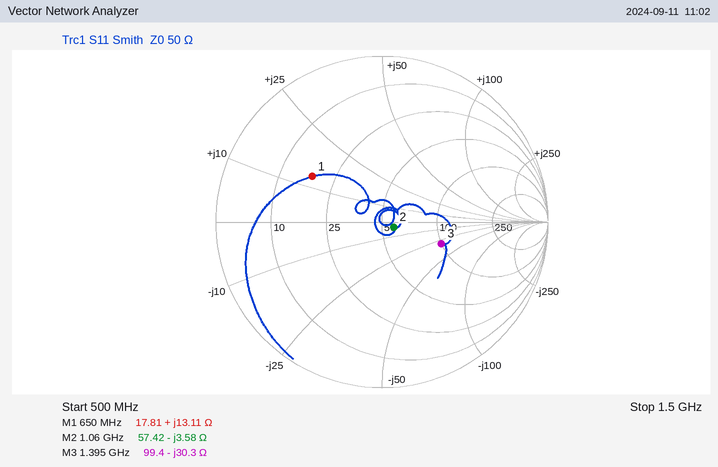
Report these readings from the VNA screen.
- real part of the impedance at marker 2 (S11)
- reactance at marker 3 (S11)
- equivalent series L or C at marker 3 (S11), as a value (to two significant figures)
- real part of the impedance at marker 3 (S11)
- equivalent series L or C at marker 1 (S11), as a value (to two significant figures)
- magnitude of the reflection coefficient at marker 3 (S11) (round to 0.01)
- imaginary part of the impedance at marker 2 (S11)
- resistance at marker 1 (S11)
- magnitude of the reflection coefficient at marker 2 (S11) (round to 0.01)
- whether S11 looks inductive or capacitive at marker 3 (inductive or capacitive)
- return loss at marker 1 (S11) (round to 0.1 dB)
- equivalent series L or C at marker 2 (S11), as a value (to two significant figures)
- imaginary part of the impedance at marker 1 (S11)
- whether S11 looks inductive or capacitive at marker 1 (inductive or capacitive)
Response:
57.42 Ω
-30.3 Ω
3.8 pF
99.4 Ω
3.2 nH
0.38
-3.58 Ω
17.81 Ω
0.08
capacitive
6.0 dB
42 pF
+13.11 Ω
inductive
